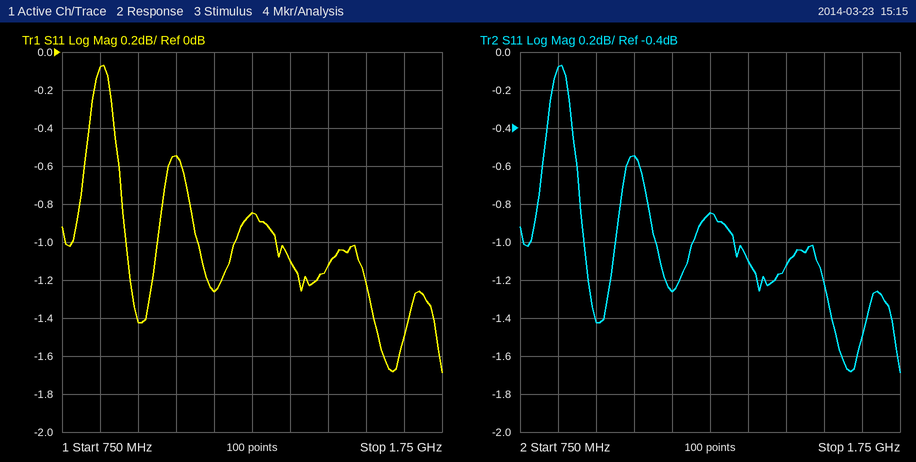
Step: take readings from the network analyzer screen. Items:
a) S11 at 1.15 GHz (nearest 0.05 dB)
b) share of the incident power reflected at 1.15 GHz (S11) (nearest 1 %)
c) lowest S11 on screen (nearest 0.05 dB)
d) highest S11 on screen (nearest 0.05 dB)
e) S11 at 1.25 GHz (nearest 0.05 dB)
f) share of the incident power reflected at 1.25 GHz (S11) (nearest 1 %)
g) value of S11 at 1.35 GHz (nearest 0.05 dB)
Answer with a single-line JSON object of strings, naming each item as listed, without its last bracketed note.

{"S11 at 1.15 GHz": "-1.25 dB", "share of the incident power reflected at 1.15 GHz (S11)": "75 %", "lowest S11 on screen": "-1.70 dB", "highest S11 on screen": "-0.05 dB", "S11 at 1.25 GHz": "-0.85 dB", "share of the incident power reflected at 1.25 GHz (S11)": "82 %", "value of S11 at 1.35 GHz": "-1.10 dB"}
